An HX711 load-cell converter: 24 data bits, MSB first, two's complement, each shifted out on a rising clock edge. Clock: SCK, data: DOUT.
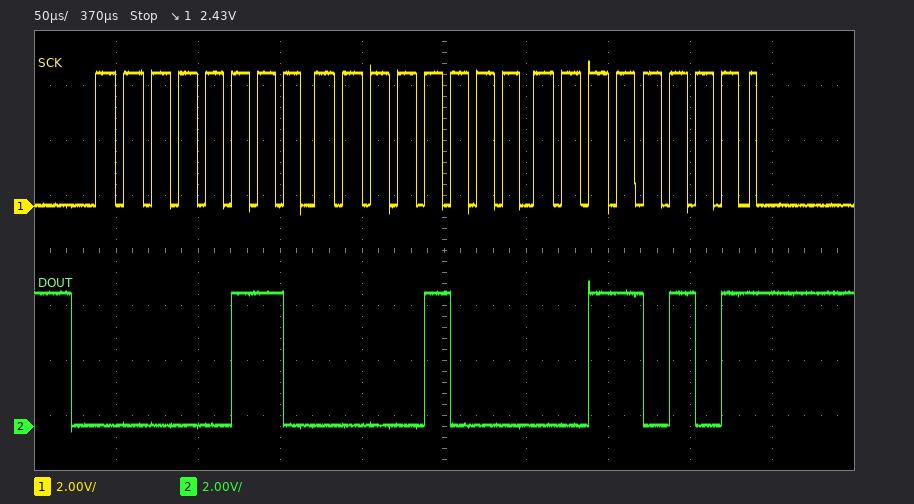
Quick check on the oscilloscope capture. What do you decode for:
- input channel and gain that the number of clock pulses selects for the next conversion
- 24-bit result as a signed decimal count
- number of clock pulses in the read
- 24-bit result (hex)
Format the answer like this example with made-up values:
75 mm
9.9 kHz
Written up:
channel A, gain 128
395317
25
0x060835
